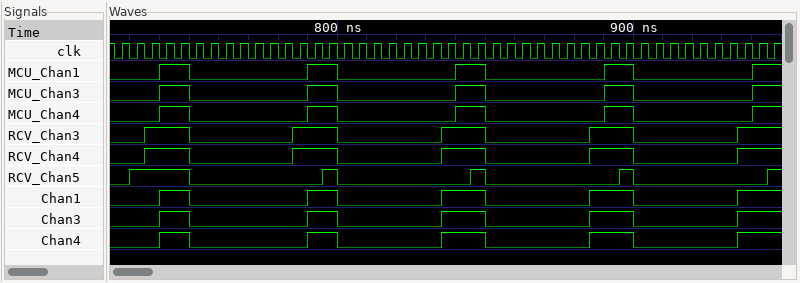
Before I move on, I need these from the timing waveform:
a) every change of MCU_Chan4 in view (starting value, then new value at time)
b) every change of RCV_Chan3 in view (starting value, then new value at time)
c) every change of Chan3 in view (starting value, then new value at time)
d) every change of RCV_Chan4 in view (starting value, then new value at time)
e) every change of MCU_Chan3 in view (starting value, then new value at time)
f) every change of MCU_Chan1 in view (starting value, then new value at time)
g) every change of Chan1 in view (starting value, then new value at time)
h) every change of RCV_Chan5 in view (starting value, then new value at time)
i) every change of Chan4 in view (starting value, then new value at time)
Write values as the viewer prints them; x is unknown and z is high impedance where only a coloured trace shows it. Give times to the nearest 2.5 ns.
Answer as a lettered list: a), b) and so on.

a) 0, 1 at 740 ns, 0 at 750 ns, 1 at 790 ns, 0 at 800 ns, 1 at 840 ns, 0 at 850 ns, 1 at 890 ns, 0 at 900 ns, 1 at 940 ns
b) 0, 1 at 735 ns, 0 at 750 ns, 1 at 785 ns, 0 at 800 ns, 1 at 835 ns, 0 at 850 ns, 1 at 885 ns, 0 at 900 ns, 1 at 935 ns
c) 0, 1 at 740 ns, 0 at 750 ns, 1 at 790 ns, 0 at 800 ns, 1 at 835 ns, 0 at 850 ns, 1 at 885 ns, 0 at 900 ns, 1 at 935 ns
d) 0, 1 at 735 ns, 0 at 750 ns, 1 at 785 ns, 0 at 800 ns, 1 at 835 ns, 0 at 850 ns, 1 at 885 ns, 0 at 900 ns, 1 at 935 ns
e) 0, 1 at 740 ns, 0 at 750 ns, 1 at 790 ns, 0 at 800 ns, 1 at 840 ns, 0 at 850 ns, 1 at 890 ns, 0 at 900 ns, 1 at 940 ns
f) 0, 1 at 740 ns, 0 at 750 ns, 1 at 790 ns, 0 at 800 ns, 1 at 840 ns, 0 at 850 ns, 1 at 890 ns, 0 at 900 ns, 1 at 940 ns
g) 0, 1 at 740 ns, 0 at 750 ns, 1 at 790 ns, 0 at 800 ns, 1 at 835 ns, 0 at 850 ns, 1 at 885 ns, 0 at 900 ns, 1 at 935 ns
h) 0, 1 at 730 ns, 0 at 750 ns, 1 at 795 ns, 0 at 800 ns, 1 at 845 ns, 0 at 850 ns, 1 at 895 ns, 0 at 900 ns, 1 at 945 ns
i) 0, 1 at 740 ns, 0 at 750 ns, 1 at 790 ns, 0 at 800 ns, 1 at 835 ns, 0 at 850 ns, 1 at 885 ns, 0 at 900 ns, 1 at 935 ns
